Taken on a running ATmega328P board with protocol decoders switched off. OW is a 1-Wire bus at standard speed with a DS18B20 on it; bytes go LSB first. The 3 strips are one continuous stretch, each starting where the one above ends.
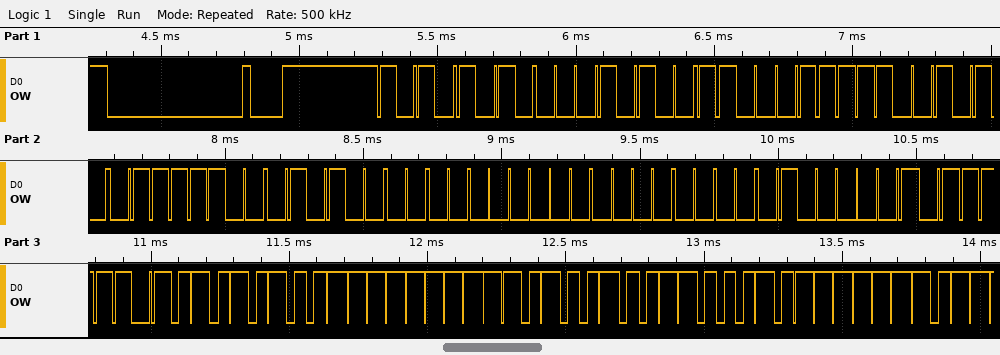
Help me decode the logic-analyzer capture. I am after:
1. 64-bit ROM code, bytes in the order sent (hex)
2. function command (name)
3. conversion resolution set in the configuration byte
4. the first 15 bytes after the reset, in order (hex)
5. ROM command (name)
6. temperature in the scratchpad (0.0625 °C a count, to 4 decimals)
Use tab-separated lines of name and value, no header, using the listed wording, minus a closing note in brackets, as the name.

64-bit ROM code, bytes in the order sent	28 E3 53 3E 0A 00 00 82
function command	Read Scratchpad
conversion resolution set in the configuration byte	12 bits
the first 15 bytes after the reset, in order	55 28 E3 53 3E 0A 00 00 82 BE 2A FF 4B 46 7F
ROM command	Match ROM
temperature in the scratchpad	-13.3750 °C
